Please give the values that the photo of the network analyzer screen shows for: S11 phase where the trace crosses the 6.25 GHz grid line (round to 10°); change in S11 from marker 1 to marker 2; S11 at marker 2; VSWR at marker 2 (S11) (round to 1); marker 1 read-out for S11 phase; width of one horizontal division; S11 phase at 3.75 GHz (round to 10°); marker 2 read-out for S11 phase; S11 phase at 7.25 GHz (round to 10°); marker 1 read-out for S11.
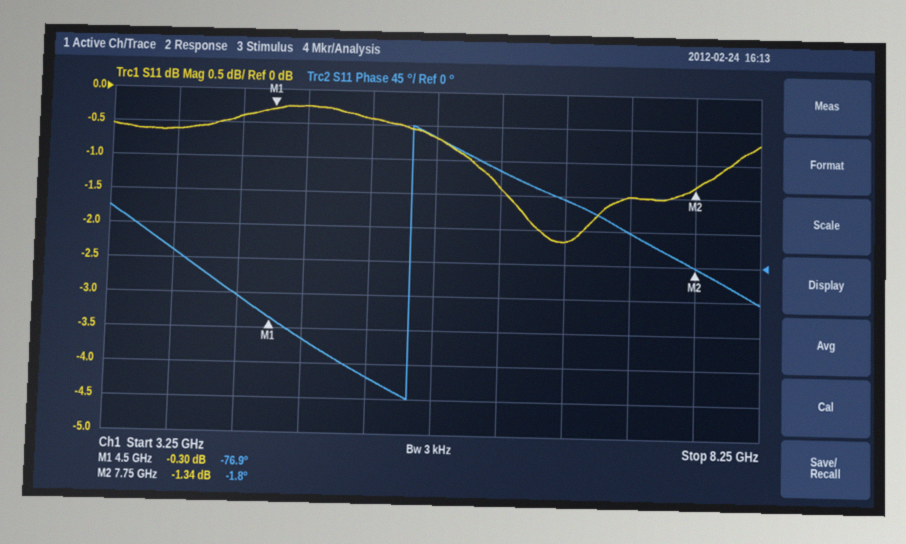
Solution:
120°
-1.04 dB
-1.34 dB
13
-76.9°
500 MHz
10°
-1.8°
40°
-0.30 dB
